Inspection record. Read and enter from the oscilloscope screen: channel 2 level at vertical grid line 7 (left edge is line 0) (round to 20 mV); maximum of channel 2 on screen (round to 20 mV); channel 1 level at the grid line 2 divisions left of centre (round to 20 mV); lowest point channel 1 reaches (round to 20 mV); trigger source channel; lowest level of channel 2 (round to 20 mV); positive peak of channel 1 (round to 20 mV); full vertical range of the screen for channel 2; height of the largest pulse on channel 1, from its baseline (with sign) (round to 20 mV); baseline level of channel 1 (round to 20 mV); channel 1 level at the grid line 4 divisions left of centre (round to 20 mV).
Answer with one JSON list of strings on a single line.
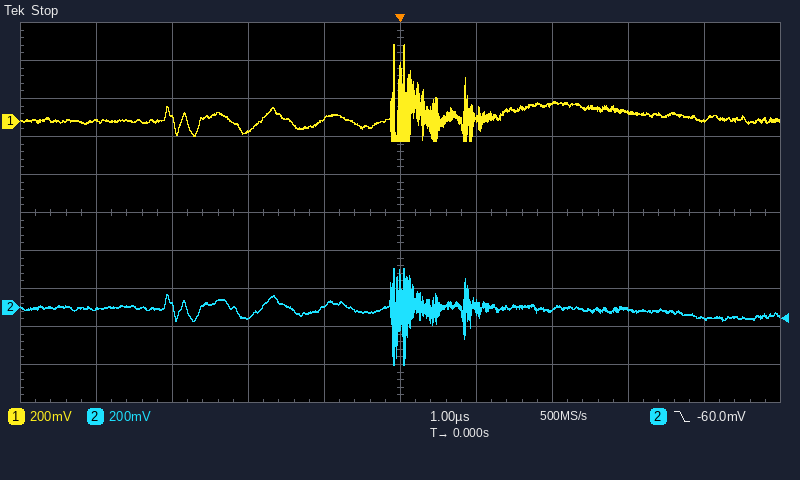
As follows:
["-20 mV", "200 mV", "-60 mV", "-100 mV", "channel 2", "-300 mV", "400 mV", "2 V", "+400 mV", "0 mV", "0 mV"]
